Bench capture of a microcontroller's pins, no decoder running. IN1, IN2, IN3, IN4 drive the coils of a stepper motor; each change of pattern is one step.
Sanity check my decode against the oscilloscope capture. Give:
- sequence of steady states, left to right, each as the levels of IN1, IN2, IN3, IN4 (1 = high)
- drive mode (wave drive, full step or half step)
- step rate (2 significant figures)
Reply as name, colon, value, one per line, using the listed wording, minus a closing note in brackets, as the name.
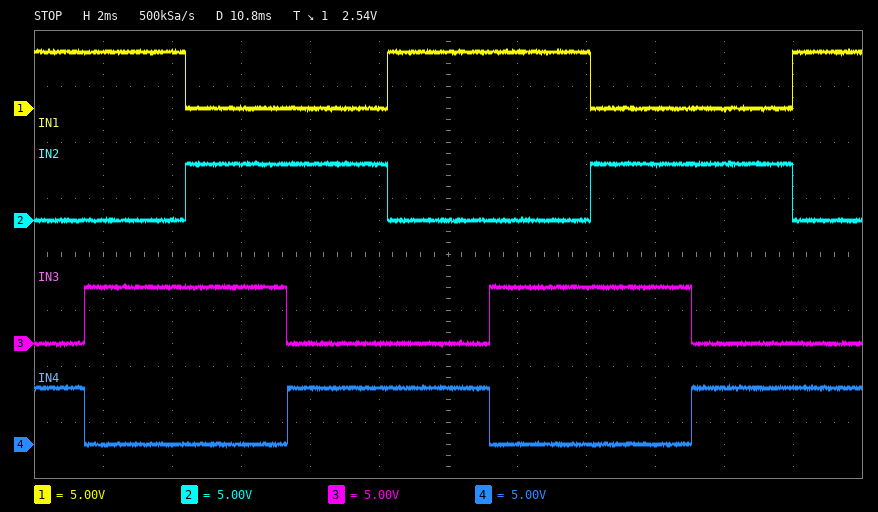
sequence of steady states, left to right, each as the levels of IN1, IN2, IN3, IN4: 1001 1010 0110 0101 1001 1010 0110 0101 1001
drive mode: full step
step rate: 340 steps/s
